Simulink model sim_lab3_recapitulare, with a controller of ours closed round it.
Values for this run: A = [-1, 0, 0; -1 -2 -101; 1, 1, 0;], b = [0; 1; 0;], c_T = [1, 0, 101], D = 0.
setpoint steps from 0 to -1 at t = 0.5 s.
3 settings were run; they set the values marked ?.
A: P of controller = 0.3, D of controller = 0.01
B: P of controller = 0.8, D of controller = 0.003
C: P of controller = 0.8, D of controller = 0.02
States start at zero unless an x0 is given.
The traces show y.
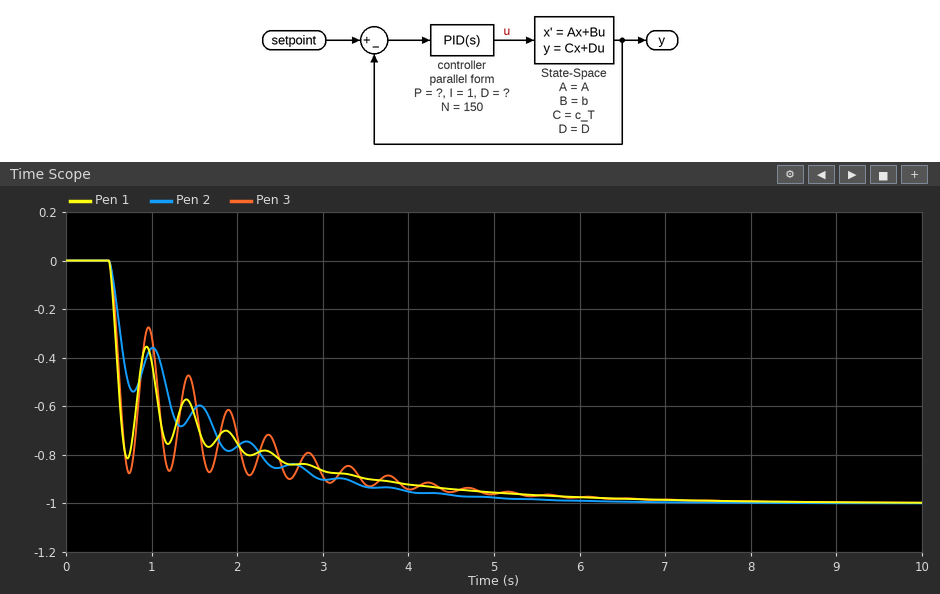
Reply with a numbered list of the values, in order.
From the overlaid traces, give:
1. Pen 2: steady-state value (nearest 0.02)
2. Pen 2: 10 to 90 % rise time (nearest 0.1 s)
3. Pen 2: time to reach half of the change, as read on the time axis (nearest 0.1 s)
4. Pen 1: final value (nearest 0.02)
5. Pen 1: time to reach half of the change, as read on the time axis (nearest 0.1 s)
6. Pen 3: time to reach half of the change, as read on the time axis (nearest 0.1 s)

1. -1.00
2. 2.4 s
3. 0.7 s
4. -1.00
5. 0.6 s
6. 0.6 s
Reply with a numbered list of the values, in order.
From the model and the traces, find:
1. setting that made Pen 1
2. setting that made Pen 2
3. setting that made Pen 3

1. C
2. A
3. B
